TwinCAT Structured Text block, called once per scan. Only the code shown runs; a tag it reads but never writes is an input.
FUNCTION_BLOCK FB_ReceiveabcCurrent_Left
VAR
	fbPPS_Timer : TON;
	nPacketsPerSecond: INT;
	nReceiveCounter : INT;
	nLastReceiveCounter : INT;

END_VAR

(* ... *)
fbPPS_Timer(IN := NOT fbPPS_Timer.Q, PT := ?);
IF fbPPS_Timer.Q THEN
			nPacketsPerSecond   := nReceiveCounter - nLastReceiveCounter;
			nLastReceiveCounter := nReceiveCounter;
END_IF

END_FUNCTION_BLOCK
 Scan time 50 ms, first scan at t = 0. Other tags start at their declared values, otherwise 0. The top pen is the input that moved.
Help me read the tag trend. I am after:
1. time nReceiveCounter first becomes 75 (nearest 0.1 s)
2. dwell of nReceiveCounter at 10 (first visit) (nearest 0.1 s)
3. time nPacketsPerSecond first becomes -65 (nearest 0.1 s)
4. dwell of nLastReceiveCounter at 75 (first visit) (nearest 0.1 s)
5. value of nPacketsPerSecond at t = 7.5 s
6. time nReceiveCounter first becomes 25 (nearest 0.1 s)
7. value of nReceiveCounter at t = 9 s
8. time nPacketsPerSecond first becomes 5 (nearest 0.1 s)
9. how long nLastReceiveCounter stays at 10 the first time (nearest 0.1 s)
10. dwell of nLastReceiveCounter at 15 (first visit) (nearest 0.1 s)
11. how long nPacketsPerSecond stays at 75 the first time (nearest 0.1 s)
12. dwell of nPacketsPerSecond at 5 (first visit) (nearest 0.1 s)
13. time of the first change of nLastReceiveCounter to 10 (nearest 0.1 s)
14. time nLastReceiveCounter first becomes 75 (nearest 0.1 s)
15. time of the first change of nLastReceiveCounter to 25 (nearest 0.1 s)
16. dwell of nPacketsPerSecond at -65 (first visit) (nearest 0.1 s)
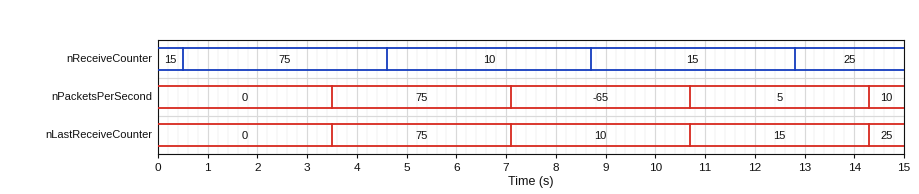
0.5 s
4.1 s
7.1 s
3.6 s
-65
12.8 s
15
10.7 s
3.6 s
3.6 s
3.6 s
3.6 s
7.1 s
3.5 s
14.3 s
3.6 s
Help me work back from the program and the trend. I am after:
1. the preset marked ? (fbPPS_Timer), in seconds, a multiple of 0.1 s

3.5 s
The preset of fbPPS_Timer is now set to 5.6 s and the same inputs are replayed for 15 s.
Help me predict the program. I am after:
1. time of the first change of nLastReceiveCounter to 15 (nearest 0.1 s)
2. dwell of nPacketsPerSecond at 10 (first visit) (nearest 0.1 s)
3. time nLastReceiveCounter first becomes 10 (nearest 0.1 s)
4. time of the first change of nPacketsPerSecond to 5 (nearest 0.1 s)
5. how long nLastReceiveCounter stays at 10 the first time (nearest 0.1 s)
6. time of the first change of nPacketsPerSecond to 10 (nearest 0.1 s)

11.3 s
5.7 s
5.6 s
11.3 s
5.7 s
5.6 s
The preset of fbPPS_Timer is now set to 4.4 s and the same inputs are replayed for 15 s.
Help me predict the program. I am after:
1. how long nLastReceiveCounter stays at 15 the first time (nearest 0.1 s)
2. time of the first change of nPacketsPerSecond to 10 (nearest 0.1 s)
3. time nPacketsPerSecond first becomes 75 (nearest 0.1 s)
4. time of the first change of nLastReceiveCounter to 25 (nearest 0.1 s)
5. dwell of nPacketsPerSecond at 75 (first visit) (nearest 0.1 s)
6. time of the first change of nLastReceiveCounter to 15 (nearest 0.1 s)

4.5 s
13.4 s
4.4 s
13.4 s
4.5 s
8.9 s
